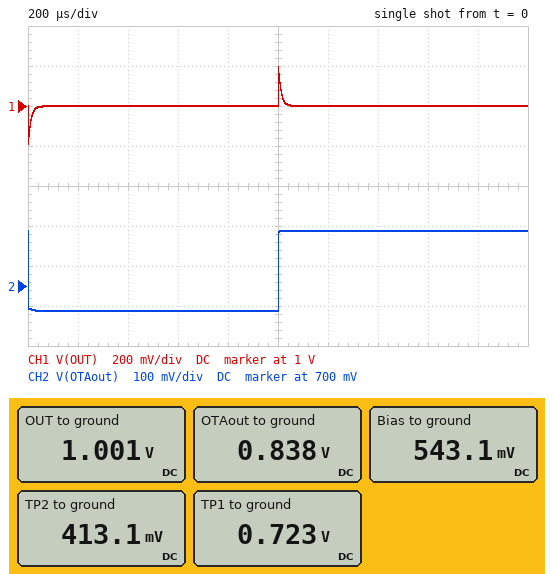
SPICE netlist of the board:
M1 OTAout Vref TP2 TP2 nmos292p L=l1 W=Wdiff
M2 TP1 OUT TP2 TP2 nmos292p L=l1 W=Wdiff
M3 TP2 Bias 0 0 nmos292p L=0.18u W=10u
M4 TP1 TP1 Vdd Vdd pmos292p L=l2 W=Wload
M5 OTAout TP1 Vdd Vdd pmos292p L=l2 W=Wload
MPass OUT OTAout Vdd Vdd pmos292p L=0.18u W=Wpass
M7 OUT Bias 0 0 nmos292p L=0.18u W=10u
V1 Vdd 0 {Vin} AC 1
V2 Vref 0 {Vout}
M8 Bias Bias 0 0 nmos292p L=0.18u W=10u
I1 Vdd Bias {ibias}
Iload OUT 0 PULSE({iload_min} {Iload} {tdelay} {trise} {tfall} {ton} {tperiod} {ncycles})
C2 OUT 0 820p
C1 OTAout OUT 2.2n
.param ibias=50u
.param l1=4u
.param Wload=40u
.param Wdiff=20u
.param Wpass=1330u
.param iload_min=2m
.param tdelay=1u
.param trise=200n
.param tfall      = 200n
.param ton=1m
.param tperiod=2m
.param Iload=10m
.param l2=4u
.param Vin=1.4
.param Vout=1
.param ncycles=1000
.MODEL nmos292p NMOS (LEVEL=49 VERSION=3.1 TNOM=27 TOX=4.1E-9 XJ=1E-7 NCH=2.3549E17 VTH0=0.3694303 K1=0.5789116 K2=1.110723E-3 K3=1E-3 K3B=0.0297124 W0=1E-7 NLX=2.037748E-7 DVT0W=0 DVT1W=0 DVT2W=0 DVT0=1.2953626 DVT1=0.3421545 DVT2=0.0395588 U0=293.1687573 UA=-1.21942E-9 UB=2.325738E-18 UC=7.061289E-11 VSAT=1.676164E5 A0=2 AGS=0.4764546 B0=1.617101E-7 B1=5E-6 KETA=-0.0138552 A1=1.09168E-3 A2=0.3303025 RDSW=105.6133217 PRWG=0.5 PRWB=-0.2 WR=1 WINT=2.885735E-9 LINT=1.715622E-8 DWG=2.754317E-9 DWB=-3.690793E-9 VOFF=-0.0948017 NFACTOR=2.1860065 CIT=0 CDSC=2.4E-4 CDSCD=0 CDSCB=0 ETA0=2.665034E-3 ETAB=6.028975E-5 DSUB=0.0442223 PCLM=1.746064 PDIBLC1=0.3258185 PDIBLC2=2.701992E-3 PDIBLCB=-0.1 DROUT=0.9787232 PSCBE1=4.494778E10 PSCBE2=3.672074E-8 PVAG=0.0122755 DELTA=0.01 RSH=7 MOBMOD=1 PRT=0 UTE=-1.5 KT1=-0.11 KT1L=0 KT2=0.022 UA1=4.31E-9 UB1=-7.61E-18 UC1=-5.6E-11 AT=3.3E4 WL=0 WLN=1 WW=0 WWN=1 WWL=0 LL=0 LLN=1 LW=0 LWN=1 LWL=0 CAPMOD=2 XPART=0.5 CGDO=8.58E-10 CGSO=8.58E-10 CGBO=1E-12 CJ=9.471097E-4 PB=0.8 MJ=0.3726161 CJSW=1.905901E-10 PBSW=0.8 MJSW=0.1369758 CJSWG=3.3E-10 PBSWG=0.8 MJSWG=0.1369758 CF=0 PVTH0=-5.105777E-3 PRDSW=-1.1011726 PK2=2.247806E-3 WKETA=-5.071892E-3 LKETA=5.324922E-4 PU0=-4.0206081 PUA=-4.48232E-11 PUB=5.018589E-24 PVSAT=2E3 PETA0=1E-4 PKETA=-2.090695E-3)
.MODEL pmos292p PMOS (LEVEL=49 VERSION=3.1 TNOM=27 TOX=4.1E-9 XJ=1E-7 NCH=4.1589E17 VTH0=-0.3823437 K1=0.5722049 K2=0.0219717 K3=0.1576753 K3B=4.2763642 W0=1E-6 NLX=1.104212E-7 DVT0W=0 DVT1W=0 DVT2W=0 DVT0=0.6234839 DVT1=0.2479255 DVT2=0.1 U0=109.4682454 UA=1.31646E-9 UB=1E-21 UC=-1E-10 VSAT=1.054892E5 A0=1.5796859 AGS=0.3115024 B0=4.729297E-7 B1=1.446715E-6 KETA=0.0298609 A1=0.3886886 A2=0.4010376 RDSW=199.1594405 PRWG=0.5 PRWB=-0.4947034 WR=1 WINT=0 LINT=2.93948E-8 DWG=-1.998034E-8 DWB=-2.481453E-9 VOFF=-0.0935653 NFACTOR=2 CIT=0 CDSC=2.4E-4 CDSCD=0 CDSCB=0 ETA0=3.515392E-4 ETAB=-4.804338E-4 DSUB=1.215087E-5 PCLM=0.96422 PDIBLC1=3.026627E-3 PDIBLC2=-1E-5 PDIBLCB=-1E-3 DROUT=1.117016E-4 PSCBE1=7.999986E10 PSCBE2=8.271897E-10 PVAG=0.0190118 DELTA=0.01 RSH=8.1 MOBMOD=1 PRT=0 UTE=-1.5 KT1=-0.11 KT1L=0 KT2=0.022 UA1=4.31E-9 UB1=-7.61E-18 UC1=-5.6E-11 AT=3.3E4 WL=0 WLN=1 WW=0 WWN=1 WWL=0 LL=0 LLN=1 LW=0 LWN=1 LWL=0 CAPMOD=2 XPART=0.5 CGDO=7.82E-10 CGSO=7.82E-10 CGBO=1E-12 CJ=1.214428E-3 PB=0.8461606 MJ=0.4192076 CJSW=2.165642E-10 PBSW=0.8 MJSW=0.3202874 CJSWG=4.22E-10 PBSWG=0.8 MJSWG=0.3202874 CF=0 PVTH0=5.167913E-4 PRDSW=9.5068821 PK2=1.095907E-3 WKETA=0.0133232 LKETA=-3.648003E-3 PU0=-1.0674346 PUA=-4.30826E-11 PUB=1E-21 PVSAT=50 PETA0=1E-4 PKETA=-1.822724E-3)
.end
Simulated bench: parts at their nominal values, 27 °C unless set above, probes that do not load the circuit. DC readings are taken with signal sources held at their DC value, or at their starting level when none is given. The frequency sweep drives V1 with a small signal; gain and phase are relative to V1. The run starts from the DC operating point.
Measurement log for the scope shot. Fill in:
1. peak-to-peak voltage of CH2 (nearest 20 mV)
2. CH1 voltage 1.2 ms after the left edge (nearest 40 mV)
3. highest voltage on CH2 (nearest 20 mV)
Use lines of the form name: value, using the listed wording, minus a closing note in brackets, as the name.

peak-to-peak voltage of CH2: 200 mV
CH1 voltage 1.2 ms after the left edge: 1.00 V
highest voltage on CH2: 840 mV
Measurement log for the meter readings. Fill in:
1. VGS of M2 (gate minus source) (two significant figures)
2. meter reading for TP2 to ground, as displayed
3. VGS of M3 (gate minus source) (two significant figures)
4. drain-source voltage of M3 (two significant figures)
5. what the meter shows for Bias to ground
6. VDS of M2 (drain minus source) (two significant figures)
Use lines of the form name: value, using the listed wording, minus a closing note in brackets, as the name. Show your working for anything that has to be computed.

VGS of M2 (gate minus source): 1.001 V - 413.1 mV = 590 mV
meter reading for TP2 to ground, as displayed: 413.1 mV
VGS of M3 (gate minus source): 543.1 mV = 540 mV
drain-source voltage of M3: 413.1 mV = 410 mV
what the meter shows for Bias to ground: 543.1 mV
VDS of M2 (drain minus source): 723 mV - 413.1 mV = 310 mV
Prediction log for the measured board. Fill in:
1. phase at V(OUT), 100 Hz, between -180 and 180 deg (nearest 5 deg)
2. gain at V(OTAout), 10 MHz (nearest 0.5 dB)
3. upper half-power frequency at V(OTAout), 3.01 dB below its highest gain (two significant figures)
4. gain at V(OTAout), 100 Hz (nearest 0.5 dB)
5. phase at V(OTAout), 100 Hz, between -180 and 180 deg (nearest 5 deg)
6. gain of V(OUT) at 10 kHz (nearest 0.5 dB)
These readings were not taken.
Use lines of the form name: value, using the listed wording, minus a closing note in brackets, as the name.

phase at V(OUT), 100 Hz, between -180 and 180 deg: 120 deg
gain at V(OTAout), 10 MHz: -6.5 dB
upper half-power frequency at V(OTAout), 3.01 dB below its highest gain: 5.1 MHz
gain at V(OTAout), 100 Hz: 0 dB
phase at V(OTAout), 100 Hz, between -180 and 180 deg: 0 deg
gain of V(OUT) at 10 kHz: -5.5 dB
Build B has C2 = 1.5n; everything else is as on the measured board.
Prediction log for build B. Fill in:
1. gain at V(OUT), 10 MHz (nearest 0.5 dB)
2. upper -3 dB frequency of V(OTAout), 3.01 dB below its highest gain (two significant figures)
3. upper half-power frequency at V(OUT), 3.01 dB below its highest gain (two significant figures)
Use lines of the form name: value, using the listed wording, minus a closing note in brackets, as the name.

gain at V(OUT), 10 MHz: -11.0 dB
upper -3 dB frequency of V(OTAout), 3.01 dB below its highest gain: 2.8 MHz
upper half-power frequency at V(OUT), 3.01 dB below its highest gain: 2.9 MHz
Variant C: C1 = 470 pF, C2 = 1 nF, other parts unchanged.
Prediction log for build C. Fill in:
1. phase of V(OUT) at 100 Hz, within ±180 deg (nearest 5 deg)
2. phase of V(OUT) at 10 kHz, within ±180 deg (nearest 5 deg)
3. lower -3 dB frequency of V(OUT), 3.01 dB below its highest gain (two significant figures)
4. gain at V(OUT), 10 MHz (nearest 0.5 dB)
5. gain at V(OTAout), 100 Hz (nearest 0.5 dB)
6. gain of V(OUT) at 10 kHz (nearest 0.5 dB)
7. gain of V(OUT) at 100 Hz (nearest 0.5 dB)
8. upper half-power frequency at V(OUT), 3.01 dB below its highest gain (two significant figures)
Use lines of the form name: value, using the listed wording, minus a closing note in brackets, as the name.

phase of V(OUT) at 100 Hz, within ±180 deg: 160 deg
phase of V(OUT) at 10 kHz, within ±180 deg: 85 deg
lower -3 dB frequency of V(OUT), 3.01 dB below its highest gain: 74 kHz
gain at V(OUT), 10 MHz: -8.0 dB
gain at V(OTAout), 100 Hz: 0 dB
gain of V(OUT) at 10 kHz: -17.5 dB
gain of V(OUT) at 100 Hz: -47.5 dB
upper half-power frequency at V(OUT), 3.01 dB below its highest gain: 4.3 MHz
